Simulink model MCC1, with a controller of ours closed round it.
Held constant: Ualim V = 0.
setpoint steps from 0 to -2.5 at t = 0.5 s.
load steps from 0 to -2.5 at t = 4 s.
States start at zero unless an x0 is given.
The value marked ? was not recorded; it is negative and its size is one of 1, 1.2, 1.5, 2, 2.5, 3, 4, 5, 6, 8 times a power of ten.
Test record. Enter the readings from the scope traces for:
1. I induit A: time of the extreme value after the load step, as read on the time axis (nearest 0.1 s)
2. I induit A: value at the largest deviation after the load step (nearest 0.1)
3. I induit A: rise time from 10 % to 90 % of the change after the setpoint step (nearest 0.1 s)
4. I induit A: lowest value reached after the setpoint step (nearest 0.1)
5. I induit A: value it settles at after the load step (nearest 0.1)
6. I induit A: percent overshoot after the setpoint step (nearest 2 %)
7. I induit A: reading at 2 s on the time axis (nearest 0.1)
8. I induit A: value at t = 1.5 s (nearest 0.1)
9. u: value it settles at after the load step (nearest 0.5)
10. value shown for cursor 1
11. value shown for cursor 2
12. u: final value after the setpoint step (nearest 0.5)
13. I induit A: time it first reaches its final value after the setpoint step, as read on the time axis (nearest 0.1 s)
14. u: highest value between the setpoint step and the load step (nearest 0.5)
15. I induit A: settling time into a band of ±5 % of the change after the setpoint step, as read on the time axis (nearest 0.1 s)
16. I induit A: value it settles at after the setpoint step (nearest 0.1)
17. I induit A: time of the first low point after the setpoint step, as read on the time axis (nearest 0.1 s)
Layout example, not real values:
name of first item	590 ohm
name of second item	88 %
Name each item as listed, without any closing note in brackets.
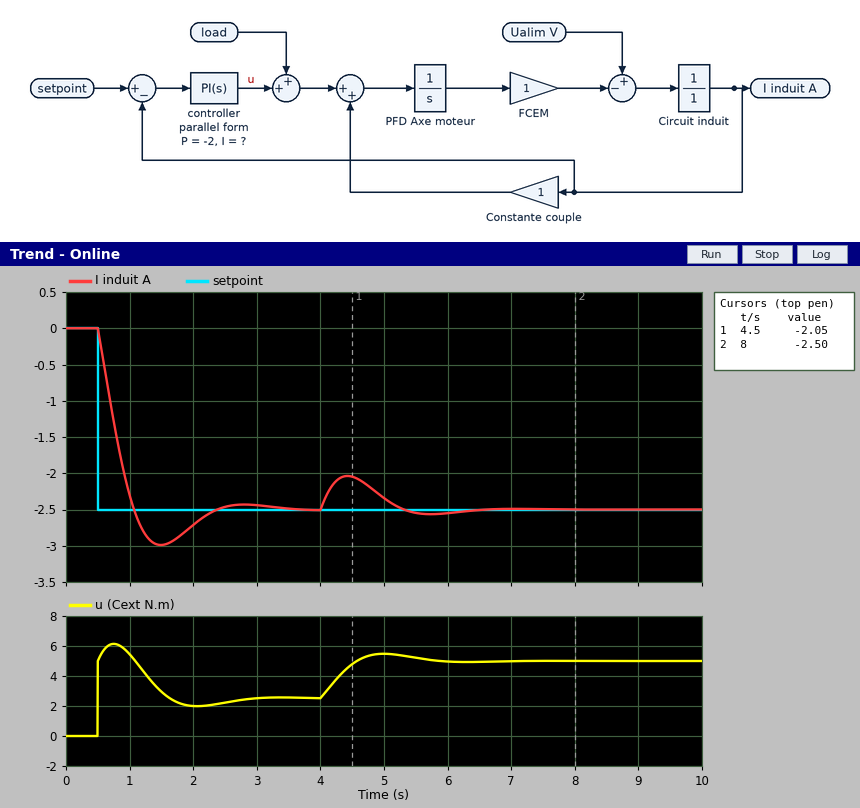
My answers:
I induit A: time of the extreme value after the load step, as read on the time axis	4.4 s
I induit A: value at the largest deviation after the load step	-2.0
I induit A: rise time from 10 % to 90 % of the change after the setpoint step	0.4 s
I induit A: lowest value reached after the setpoint step	-3.0
I induit A: value it settles at after the load step	-2.5
I induit A: percent overshoot after the setpoint step	20 %
I induit A: reading at 2 s on the time axis	-2.7
I induit A: value at t = 1.5 s	-3.0
u: value it settles at after the load step	5.0
value shown for cursor 1	-2.05
value shown for cursor 2	-2.50
u: final value after the setpoint step	2.5
I induit A: time it first reaches its final value after the setpoint step, as read on the time axis	1.1 s
u: highest value between the setpoint step and the load step	6.0
I induit A: settling time into a band of ±5 % of the change after the setpoint step, as read on the time axis	2.1 s
I induit A: value it settles at after the setpoint step	-2.5
I induit A: time of the first low point after the setpoint step, as read on the time axis	1.5 s
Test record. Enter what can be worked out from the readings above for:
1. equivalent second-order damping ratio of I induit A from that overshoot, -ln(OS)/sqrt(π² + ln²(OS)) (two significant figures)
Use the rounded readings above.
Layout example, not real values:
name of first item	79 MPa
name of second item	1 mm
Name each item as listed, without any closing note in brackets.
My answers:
equivalent second-order damping ratio of I induit A from that overshoot, -ln(OS)/sqrt(π² + ln²(OS))	0.46
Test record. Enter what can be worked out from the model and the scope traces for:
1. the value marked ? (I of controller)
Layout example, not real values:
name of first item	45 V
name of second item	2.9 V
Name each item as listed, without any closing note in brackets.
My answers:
the value marked ?	-8
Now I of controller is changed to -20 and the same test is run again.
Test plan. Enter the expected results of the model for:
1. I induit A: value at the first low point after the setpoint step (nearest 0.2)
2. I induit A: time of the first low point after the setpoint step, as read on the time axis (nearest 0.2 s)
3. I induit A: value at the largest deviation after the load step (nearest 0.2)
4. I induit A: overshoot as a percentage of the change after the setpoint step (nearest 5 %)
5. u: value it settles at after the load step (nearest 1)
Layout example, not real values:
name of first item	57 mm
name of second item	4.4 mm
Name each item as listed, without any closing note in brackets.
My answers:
I induit A: value at the first low point after the setpoint step	-3.4
I induit A: time of the first low point after the setpoint step, as read on the time axis	1.2 s
I induit A: value at the largest deviation after the load step	-2.2
I induit A: overshoot as a percentage of the change after the setpoint step	35 %
u: value it settles at after the load step	5
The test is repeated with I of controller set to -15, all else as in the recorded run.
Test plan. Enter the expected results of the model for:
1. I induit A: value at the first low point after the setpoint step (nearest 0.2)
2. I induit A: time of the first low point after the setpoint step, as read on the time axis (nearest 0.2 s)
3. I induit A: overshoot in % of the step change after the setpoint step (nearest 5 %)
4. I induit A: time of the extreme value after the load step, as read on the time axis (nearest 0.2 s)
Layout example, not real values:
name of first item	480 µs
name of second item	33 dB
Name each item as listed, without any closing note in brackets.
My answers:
I induit A: value at the first low point after the setpoint step	-3.2
I induit A: time of the first low point after the setpoint step, as read on the time axis	1.2 s
I induit A: overshoot in % of the step change after the setpoint step	30 %
I induit A: time of the extreme value after the load step, as read on the time axis	4.4 s
